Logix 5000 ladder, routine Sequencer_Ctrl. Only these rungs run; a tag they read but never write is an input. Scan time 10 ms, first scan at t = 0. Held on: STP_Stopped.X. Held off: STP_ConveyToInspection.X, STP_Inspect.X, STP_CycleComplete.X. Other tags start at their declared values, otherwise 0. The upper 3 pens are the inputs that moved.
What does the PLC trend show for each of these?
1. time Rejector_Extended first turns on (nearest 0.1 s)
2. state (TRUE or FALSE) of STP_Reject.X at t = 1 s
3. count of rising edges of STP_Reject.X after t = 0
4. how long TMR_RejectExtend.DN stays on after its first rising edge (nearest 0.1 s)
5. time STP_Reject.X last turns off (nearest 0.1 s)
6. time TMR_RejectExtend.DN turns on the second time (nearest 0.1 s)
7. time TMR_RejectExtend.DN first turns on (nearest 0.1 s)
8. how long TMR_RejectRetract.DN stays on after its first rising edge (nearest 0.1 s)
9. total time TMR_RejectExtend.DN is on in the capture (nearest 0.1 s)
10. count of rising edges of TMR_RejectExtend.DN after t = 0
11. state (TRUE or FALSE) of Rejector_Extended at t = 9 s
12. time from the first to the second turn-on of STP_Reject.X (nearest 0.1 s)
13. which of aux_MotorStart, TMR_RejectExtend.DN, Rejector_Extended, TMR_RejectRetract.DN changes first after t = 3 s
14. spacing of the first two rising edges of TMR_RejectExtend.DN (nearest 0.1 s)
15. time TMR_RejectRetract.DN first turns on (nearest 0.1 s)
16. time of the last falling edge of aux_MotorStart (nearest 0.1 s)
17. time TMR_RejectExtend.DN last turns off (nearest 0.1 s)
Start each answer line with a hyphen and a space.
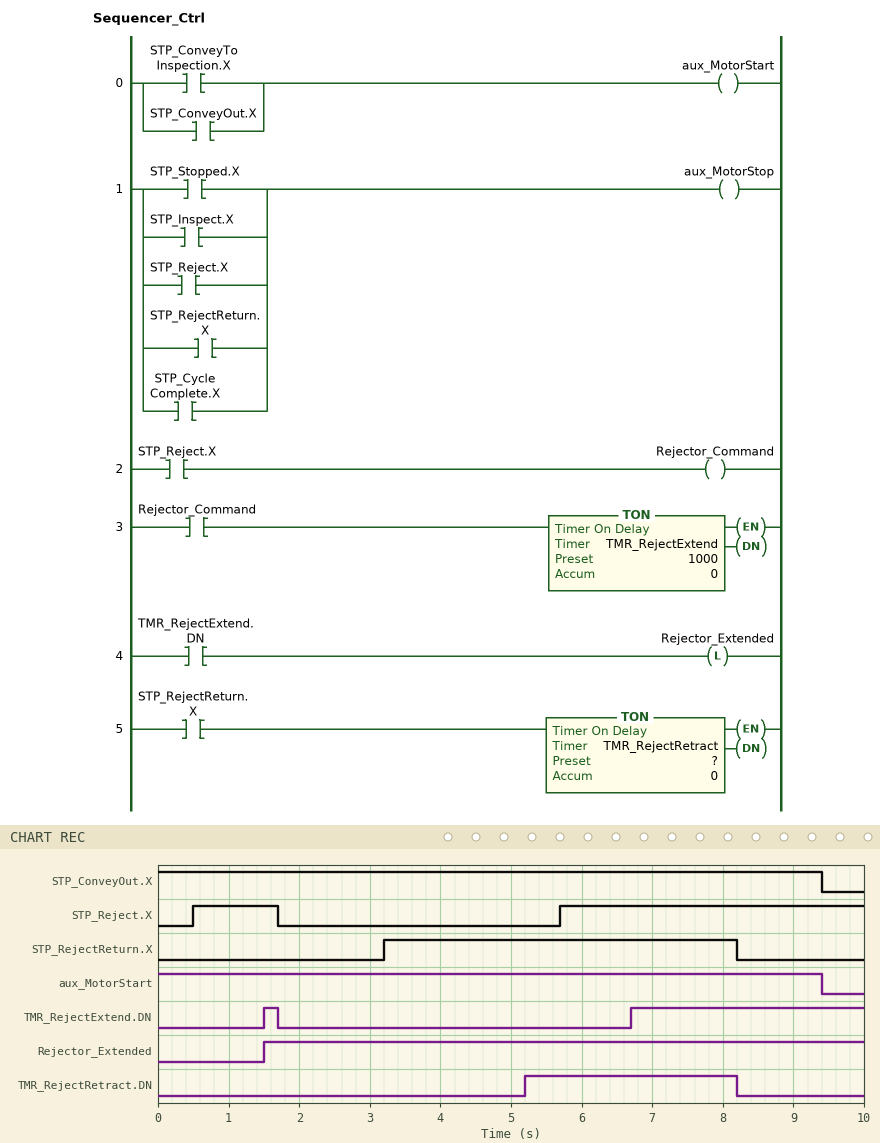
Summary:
- 1.5 s
- TRUE
- 2
- 0.2 s
- 1.7 s
- 6.7 s
- 1.5 s
- 3.0 s
- 3.5 s
- 2
- TRUE
- 5.2 s
- TMR_RejectRetract.DN
- 5.2 s
- 5.2 s
- 9.4 s
- 1.7 s
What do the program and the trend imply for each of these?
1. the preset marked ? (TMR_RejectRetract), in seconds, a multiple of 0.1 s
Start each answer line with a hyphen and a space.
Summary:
- 2.0 s
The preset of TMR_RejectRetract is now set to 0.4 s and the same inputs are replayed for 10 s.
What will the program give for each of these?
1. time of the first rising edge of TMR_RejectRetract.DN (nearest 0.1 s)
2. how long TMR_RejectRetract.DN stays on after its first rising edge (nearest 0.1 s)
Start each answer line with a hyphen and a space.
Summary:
- 3.6 s
- 4.6 s
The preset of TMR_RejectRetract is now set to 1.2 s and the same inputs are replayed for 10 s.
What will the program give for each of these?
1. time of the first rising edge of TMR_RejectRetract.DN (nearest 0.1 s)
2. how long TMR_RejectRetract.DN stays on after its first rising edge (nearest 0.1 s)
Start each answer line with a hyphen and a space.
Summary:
- 4.4 s
- 3.8 s
